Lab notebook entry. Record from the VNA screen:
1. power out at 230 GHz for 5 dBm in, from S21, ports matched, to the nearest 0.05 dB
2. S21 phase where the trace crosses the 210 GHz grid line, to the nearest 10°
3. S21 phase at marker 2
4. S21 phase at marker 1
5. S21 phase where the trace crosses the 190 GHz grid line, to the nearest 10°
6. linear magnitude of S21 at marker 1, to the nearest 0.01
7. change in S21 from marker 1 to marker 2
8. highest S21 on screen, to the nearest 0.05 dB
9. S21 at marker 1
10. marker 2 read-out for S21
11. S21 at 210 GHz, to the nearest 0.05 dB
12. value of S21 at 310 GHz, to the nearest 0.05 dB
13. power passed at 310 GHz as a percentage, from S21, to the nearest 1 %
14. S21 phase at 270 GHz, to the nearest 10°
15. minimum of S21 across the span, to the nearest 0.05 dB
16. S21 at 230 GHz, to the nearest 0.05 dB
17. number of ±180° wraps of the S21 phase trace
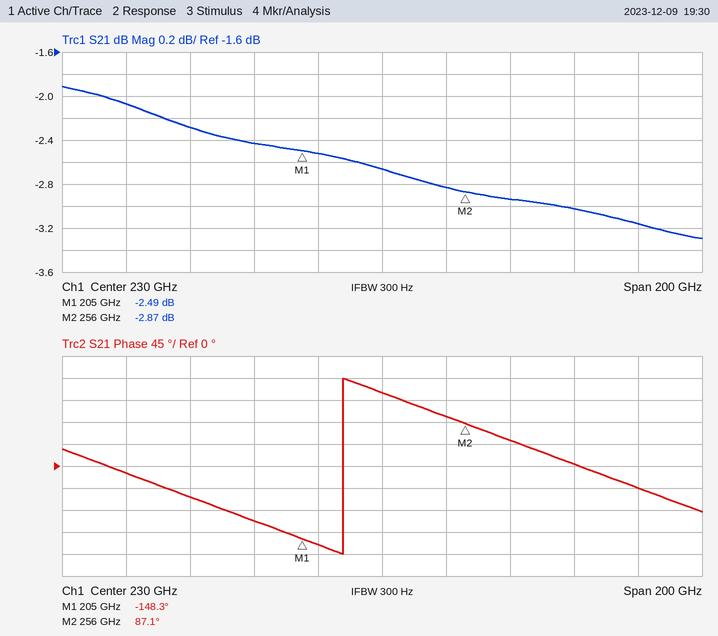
2.35 dBm
-160°
87.1°
-148.3°
-110°
0.75
-0.38 dB
-1.90 dB
-2.49 dB
-2.87 dB
-2.50 dB
-3.15 dB
48 %
50°
-3.30 dB
-2.65 dB
1
